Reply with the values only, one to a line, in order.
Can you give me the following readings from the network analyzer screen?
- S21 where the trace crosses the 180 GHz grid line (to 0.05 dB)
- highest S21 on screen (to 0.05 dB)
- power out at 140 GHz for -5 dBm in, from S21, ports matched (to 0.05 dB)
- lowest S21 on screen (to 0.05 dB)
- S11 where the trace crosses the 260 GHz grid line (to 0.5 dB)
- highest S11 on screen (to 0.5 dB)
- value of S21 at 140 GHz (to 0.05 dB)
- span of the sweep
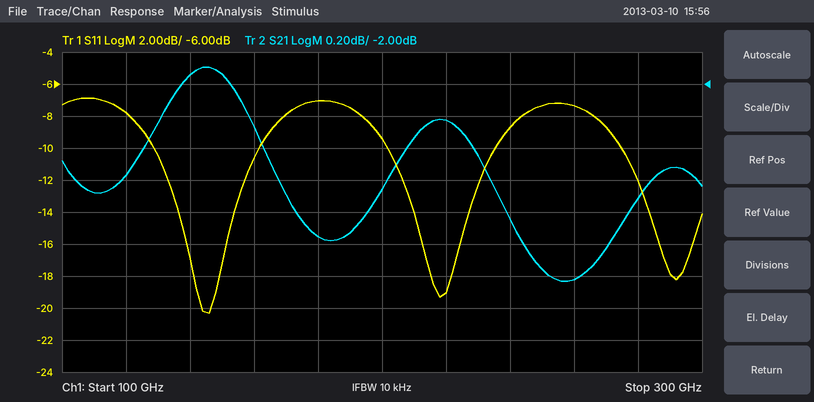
-2.95 dB
-1.90 dB
-6.95 dBm
-3.25 dB
-7.5 dB
-7.0 dB
-1.95 dB
200 GHz
